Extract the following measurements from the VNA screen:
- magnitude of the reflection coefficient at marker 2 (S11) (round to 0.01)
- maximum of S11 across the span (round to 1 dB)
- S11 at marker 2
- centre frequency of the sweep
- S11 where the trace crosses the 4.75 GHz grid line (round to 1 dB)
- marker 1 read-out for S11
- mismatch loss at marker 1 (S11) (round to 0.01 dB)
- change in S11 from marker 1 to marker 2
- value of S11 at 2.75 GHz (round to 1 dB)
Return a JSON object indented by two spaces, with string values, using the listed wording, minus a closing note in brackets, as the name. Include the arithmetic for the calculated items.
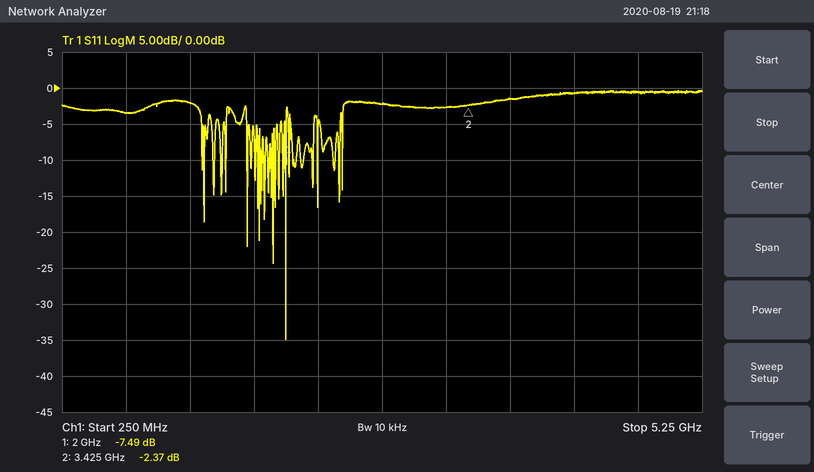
{
  "magnitude of the reflection coefficient at marker 2 (S11)": "10^(-2.37/20) ≈ 0.76",
  "maximum of S11 across the span": "0 dB",
  "S11 at marker 2": "-2.37 dB",
  "centre frequency of the sweep": "2.75 GHz",
  "S11 where the trace crosses the 4.75 GHz grid line": "-1 dB",
  "marker 1 read-out for S11": "-7.49 dB",
  "mismatch loss at marker 1 (S11)": "−10 log10(1 − 10^(-7.49/10)) ≈ 0.85 dB",
  "change in S11 from marker 1 to marker 2": "-2.37 − (-7.49) = 5.12 dB",
  "value of S11 at 2.75 GHz": "-2 dB"
}
